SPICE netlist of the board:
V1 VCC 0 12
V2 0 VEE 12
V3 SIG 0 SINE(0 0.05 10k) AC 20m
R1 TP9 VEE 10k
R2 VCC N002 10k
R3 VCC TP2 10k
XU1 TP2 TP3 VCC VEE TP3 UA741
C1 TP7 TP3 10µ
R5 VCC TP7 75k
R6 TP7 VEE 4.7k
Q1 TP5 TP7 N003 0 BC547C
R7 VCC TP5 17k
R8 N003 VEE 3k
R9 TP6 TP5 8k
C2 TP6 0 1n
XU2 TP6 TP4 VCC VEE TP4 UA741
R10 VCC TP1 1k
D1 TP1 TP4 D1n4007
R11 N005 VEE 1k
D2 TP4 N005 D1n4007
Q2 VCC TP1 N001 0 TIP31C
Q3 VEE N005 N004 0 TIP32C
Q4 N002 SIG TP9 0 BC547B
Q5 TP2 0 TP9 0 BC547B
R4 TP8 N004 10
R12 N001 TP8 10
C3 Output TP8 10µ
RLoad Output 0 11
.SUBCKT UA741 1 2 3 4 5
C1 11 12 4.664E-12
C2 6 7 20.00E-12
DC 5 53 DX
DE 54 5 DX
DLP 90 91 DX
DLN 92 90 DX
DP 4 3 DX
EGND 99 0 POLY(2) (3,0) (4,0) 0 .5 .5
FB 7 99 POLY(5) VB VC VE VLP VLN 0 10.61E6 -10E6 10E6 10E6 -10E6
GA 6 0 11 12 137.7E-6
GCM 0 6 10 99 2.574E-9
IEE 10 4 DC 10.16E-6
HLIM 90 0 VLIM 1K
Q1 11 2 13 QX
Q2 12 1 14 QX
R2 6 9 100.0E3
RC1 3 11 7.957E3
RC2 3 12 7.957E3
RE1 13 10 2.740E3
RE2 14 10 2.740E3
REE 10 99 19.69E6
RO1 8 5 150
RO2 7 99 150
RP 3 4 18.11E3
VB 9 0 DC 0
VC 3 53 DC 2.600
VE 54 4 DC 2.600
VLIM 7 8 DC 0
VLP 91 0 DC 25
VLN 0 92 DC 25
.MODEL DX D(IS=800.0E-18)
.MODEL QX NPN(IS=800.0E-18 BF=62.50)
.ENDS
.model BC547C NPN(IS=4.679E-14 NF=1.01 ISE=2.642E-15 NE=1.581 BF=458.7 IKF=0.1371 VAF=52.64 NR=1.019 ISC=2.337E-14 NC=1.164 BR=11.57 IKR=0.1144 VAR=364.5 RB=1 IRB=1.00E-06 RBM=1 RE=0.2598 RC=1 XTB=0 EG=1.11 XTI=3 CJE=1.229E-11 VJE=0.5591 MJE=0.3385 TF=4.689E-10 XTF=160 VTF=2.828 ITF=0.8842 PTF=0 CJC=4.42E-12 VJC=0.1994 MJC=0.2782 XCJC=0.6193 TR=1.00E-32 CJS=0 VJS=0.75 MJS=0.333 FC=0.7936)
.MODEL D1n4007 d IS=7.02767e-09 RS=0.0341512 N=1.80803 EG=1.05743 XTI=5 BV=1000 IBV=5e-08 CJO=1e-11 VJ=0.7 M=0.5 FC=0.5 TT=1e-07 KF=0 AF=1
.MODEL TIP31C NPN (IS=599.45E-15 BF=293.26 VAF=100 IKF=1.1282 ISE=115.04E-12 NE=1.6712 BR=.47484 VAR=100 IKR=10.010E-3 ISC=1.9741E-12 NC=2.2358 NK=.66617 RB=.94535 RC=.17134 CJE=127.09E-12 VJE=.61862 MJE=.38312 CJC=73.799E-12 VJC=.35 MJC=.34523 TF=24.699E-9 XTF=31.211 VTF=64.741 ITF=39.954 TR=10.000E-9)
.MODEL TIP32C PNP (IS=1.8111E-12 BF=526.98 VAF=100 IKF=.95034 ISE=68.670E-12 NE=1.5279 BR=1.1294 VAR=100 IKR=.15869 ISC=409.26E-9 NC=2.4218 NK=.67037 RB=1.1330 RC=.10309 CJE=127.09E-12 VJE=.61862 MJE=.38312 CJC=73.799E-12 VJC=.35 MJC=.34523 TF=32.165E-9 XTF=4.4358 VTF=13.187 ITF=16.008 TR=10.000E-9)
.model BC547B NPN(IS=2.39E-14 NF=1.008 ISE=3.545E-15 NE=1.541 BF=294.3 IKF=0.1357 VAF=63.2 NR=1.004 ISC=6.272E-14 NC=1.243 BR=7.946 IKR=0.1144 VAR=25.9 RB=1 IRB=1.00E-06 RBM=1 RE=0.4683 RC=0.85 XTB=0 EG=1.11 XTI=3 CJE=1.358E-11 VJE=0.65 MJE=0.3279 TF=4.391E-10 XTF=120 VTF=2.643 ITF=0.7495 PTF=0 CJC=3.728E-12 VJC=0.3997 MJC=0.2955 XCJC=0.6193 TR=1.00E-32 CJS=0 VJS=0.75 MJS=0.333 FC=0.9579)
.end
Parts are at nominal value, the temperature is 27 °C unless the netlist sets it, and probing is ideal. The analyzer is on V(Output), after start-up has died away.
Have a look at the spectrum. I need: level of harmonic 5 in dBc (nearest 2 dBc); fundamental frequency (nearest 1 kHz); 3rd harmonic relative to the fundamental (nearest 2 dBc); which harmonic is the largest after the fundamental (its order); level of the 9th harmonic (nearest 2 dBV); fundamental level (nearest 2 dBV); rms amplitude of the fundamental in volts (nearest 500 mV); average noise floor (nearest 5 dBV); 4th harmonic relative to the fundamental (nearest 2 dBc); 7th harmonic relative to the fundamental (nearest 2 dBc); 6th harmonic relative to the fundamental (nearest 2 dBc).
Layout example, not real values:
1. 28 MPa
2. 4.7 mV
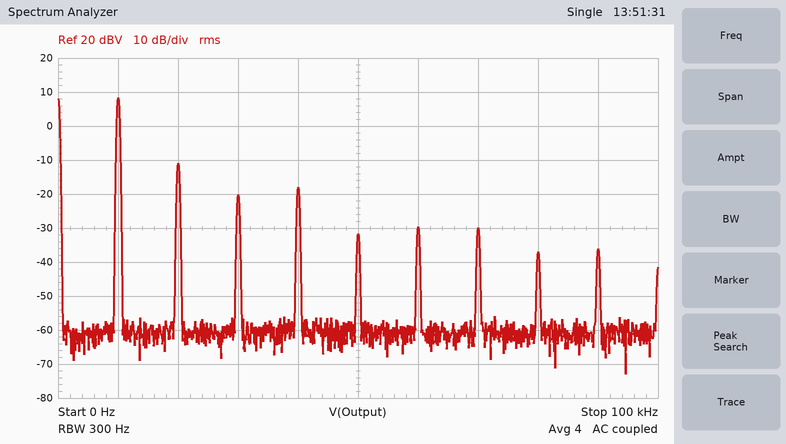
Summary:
1. -40 dBc
2. 10 kHz
3. -28 dBc
4. 2
5. -36 dBV
6. 8 dBV
7. 2.5 V
8. -60 dBV
9. -26 dBc
10. -38 dBc
11. -38 dBc
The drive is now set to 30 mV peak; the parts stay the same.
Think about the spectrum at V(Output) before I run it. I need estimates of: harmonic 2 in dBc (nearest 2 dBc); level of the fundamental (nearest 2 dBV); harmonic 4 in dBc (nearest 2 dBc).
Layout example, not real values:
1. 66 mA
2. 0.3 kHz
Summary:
1. -16 dBc
2. 6 dBV
3. -36 dBc
